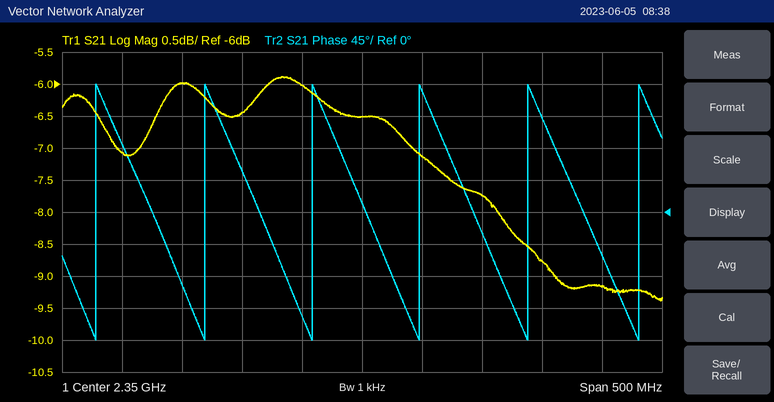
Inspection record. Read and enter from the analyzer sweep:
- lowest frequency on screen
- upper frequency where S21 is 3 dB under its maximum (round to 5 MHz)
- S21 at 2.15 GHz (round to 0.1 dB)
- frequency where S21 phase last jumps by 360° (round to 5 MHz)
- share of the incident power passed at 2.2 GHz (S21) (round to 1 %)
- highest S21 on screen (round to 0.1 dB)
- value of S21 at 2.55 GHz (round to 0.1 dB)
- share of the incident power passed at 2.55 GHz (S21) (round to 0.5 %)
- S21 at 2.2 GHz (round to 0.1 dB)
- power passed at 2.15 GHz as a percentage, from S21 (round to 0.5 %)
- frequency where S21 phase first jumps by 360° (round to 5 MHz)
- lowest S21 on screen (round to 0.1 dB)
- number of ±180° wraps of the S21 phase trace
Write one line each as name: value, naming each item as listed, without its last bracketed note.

lowest frequency on screen: 2.1 GHz
upper frequency where S21 is 3 dB under its maximum: 2.505 GHz
S21 at 2.15 GHz: -7.1 dB
frequency where S21 phase last jumps by 360°: 2.580 GHz
share of the incident power passed at 2.2 GHz (S21): 25 %
highest S21 on screen: -5.9 dB
value of S21 at 2.55 GHz: -9.2 dB
share of the incident power passed at 2.55 GHz (S21): 12.0 %
S21 at 2.2 GHz: -6.0 dB
power passed at 2.15 GHz as a percentage, from S21: 19.5 %
frequency where S21 phase first jumps by 360°: 2.130 GHz
lowest S21 on screen: -9.4 dB
number of ±180° wraps of the S21 phase trace: 6
